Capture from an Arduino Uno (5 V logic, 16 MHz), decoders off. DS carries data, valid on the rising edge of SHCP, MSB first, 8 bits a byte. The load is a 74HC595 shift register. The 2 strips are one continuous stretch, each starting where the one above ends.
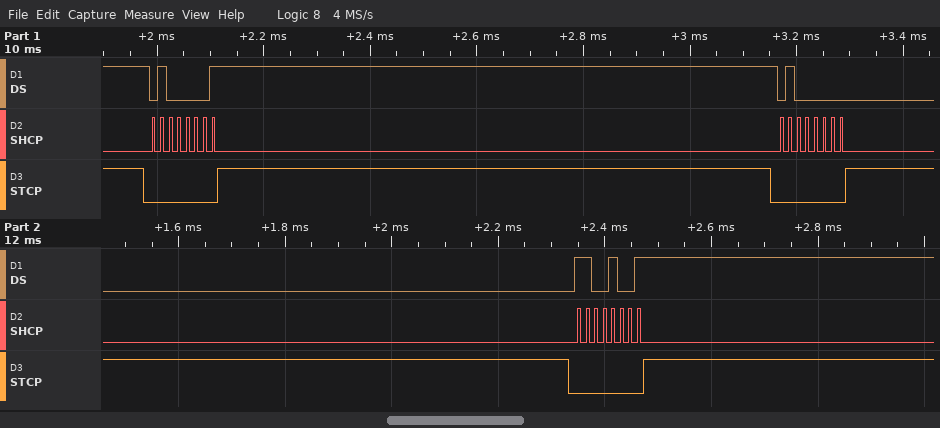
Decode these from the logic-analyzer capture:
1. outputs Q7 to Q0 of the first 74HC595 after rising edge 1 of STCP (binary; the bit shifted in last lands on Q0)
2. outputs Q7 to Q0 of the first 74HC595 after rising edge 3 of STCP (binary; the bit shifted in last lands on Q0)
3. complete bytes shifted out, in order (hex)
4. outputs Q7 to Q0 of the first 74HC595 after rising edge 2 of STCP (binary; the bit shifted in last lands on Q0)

01000001
11001001
41 40 C9
01000000
